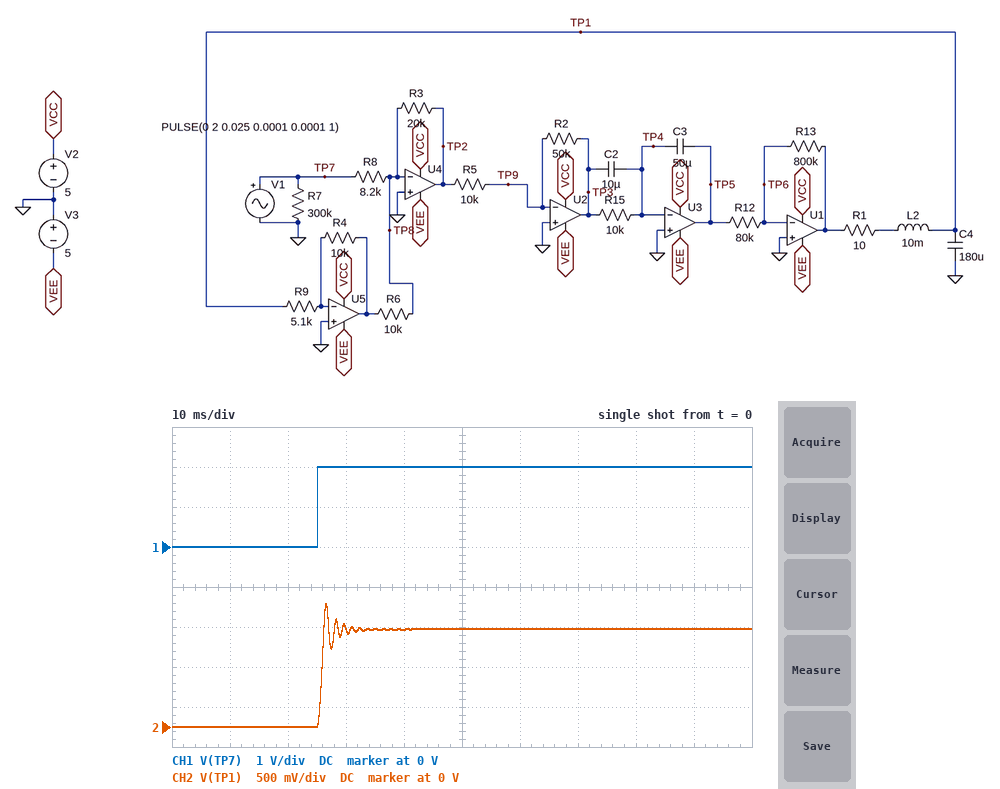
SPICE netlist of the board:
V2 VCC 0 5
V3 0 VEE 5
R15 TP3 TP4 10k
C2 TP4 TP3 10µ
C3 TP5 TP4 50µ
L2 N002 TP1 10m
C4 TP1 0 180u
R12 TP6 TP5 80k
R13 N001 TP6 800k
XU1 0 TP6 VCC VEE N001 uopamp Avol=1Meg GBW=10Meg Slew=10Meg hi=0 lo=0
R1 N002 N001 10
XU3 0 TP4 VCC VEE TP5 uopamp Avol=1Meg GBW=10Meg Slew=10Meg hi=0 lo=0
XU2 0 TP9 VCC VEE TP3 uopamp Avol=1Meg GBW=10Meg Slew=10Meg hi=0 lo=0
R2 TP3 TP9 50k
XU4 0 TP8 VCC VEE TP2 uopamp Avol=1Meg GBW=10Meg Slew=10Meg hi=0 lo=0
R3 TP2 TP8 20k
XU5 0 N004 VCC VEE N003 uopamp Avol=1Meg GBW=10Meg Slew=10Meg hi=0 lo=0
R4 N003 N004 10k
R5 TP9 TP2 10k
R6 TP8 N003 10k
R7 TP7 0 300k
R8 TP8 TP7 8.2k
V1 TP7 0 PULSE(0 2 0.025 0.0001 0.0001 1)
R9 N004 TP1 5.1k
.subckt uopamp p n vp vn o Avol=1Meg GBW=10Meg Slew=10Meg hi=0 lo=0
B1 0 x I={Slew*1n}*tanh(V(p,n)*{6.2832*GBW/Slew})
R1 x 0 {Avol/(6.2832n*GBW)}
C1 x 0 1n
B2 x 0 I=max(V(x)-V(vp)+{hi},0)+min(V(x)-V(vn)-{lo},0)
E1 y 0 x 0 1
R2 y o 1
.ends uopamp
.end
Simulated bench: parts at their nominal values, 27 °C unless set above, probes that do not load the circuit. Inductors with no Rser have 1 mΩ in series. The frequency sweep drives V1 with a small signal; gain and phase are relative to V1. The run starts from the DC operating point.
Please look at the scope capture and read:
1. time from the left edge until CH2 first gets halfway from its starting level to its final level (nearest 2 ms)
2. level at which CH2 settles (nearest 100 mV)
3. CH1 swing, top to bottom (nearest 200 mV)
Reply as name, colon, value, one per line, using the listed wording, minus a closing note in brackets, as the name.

time from the left edge until CH2 first gets halfway from its starting level to its final level: 26 ms
level at which CH2 settles: 1.2 V
CH1 swing, top to bottom: 2.0 V
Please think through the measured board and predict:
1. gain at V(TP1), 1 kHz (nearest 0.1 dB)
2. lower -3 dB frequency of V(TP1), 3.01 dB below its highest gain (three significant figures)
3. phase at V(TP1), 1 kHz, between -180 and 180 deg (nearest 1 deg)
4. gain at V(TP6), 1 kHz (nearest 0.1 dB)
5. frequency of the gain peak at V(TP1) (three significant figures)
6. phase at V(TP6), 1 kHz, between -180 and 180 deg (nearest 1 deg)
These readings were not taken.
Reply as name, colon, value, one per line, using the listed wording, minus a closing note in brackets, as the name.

gain at V(TP1), 1 kHz: -2.6 dB
lower -3 dB frequency of V(TP1), 3.01 dB below its highest gain: 661 Hz
phase at V(TP1), 1 kHz, between -180 and 180 deg: -160 deg
gain at V(TP6), 1 kHz: -45.5 dB
frequency of the gain peak at V(TP1): 744 Hz
phase at V(TP6), 1 kHz, between -180 and 180 deg: -81 deg
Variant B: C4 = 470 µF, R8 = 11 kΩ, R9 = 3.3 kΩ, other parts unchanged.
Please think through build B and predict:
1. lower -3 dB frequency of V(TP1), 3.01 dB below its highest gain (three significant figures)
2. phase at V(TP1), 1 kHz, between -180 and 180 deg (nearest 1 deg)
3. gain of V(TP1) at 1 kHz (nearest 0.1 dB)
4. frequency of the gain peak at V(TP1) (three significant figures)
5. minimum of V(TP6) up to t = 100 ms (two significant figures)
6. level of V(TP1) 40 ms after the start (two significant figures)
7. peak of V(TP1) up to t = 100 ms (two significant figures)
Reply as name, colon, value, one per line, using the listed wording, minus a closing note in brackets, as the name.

lower -3 dB frequency of V(TP1), 3.01 dB below its highest gain: 480 Hz
phase at V(TP1), 1 kHz, between -180 and 180 deg: -167 deg
gain of V(TP1) at 1 kHz: -16.9 dB
frequency of the gain peak at V(TP1): 565 Hz
minimum of V(TP6) up to t = 100 ms: -490 mV
level of V(TP1) 40 ms after the start: 590 mV
peak of V(TP1) up to t = 100 ms: 750 mV
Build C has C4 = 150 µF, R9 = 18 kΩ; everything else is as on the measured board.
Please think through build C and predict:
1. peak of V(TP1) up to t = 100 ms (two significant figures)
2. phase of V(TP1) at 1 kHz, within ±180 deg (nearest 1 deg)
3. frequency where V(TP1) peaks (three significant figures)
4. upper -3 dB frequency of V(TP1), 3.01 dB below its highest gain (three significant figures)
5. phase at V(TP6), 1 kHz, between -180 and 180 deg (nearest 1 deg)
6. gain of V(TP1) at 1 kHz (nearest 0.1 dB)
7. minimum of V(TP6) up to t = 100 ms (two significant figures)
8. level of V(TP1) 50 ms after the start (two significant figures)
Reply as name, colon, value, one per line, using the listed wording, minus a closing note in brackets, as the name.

peak of V(TP1) up to t = 100 ms: 4.4 V
phase of V(TP1) at 1 kHz, within ±180 deg: -169 deg
frequency where V(TP1) peaks: 438 Hz
upper -3 dB frequency of V(TP1), 3.01 dB below its highest gain: 512 Hz
phase at V(TP6), 1 kHz, between -180 and 180 deg: -90 deg
gain of V(TP1) at 1 kHz: -5.9 dB
minimum of V(TP6) up to t = 100 ms: -500 mV
level of V(TP1) 50 ms after the start: 4.1 V
